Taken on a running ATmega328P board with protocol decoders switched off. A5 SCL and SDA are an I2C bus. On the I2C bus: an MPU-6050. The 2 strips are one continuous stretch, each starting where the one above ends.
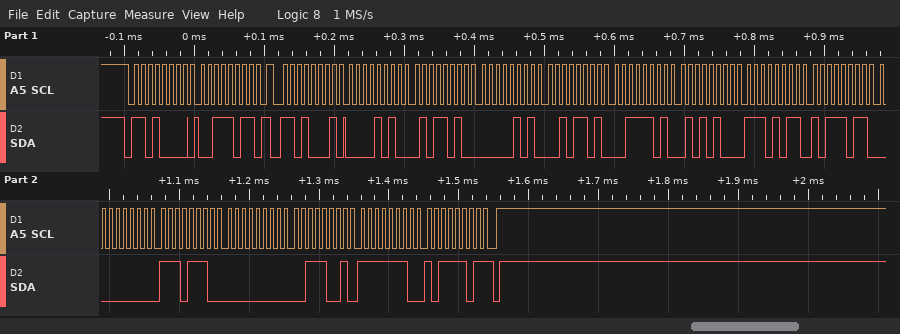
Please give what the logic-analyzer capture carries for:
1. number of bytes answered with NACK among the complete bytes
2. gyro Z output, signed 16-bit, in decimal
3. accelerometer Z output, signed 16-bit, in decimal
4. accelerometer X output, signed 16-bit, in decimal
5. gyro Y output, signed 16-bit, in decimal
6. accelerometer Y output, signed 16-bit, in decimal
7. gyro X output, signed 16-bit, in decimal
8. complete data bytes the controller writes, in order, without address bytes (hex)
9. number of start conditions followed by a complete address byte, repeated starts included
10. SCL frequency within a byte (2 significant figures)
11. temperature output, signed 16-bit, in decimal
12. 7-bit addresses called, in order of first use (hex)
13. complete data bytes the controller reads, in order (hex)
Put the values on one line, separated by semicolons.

1; -323; 15700; 2650; 57; 1325; 238; 3B; 2; 100 kHz; -5189; 0x68; 0A 5A 05 2D 3D 54 EB BB 00 EE 00 39 FE BD
